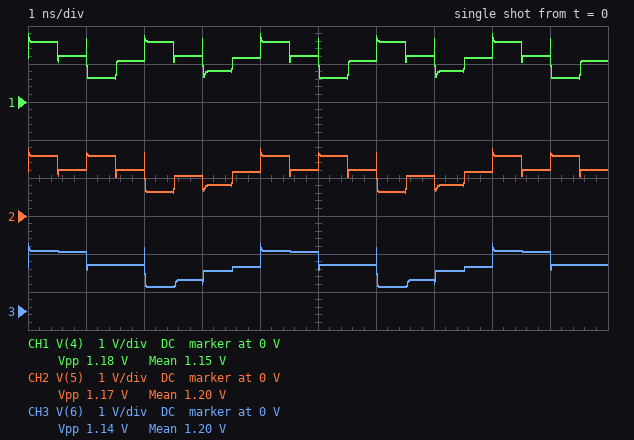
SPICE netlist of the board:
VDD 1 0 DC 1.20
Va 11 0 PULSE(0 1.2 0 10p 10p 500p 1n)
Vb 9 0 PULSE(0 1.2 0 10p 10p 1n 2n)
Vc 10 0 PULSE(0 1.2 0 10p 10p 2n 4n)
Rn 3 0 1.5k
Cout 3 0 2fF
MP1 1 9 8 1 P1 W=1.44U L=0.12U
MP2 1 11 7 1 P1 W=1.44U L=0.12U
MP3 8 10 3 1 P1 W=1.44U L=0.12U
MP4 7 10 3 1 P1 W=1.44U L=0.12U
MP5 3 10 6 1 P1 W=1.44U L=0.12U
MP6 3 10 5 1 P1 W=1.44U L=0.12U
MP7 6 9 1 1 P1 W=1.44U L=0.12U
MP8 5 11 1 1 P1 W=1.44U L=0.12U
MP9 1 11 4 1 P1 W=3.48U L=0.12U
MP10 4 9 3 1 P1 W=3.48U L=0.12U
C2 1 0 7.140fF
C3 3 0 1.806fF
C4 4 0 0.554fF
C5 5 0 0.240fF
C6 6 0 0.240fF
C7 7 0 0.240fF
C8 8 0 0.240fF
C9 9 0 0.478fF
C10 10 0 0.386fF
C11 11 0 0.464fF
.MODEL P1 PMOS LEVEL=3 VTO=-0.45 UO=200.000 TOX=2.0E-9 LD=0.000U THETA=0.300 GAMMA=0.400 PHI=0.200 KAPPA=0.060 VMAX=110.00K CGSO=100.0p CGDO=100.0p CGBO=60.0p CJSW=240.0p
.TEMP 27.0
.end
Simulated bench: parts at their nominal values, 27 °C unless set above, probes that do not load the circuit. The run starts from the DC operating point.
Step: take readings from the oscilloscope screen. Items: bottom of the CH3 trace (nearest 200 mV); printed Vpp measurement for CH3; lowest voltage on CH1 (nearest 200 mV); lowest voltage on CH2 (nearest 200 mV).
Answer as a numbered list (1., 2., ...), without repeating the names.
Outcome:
1. 600 mV
2. 1.14 V
3. 600 mV
4. 600 mV
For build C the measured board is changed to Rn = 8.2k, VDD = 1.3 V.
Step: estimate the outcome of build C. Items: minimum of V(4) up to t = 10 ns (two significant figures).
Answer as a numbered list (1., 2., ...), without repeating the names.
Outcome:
1. 620 mV
